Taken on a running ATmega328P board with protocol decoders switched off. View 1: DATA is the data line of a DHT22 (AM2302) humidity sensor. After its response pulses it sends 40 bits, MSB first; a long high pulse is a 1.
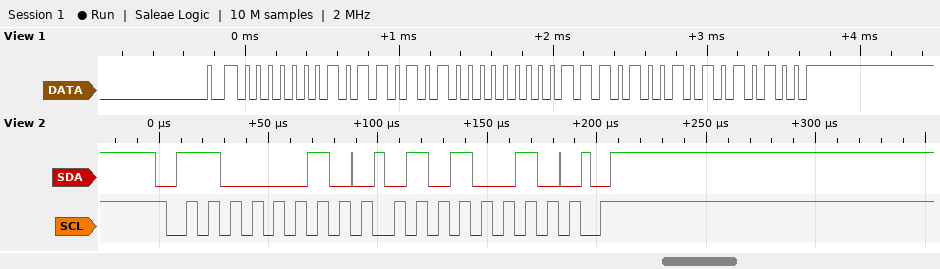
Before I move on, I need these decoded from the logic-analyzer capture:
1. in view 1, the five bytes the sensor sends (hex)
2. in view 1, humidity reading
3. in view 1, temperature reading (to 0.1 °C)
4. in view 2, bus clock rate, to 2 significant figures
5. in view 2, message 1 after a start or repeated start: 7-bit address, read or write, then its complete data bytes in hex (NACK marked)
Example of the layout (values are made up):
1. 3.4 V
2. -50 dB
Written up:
1. 01 6A 00 E9 54
2. 36.2 %
3. 23.3 °C
4. 100 kHz
5. 0x61 write: 52
